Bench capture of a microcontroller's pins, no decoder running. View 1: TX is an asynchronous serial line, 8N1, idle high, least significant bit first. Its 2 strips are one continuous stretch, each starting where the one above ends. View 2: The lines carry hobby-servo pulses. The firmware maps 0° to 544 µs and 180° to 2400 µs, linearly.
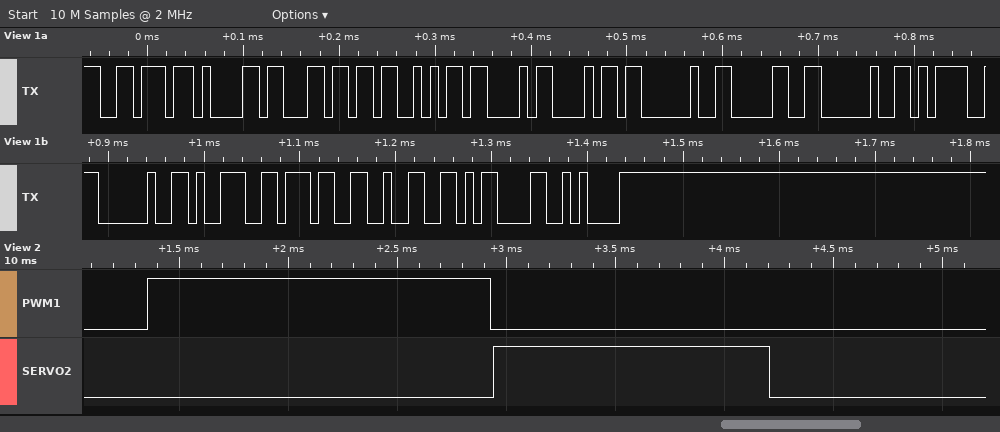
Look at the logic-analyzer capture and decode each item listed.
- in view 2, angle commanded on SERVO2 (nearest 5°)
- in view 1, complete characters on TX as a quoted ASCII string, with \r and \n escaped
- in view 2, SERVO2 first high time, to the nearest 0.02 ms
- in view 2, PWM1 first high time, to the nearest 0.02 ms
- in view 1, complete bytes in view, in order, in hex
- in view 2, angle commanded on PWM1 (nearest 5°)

70°
"valSCh 0 = 972\r\n"
1.26 ms
1.58 ms
76 61 6C 53 43 68 20 30 20 3D 20 39 37 32 0D 0A
100°
